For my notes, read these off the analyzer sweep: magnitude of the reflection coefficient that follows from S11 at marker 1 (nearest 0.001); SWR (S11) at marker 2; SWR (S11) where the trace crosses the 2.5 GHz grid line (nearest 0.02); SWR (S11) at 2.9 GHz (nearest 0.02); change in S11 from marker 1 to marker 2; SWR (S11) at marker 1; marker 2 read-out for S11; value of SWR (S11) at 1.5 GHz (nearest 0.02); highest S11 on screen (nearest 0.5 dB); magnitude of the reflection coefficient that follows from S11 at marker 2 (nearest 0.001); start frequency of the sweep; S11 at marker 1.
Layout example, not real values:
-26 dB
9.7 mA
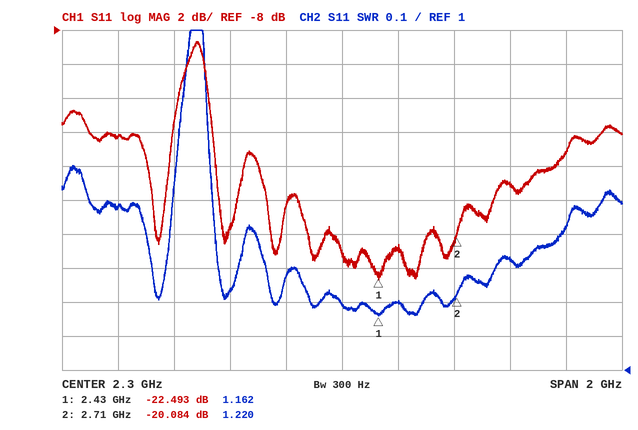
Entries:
0.075
1.220
1.20
1.32
2.409 dB
1.162
-20.084 dB
1.48
-8.5 dB
0.099
1.3 GHz
-22.493 dB
